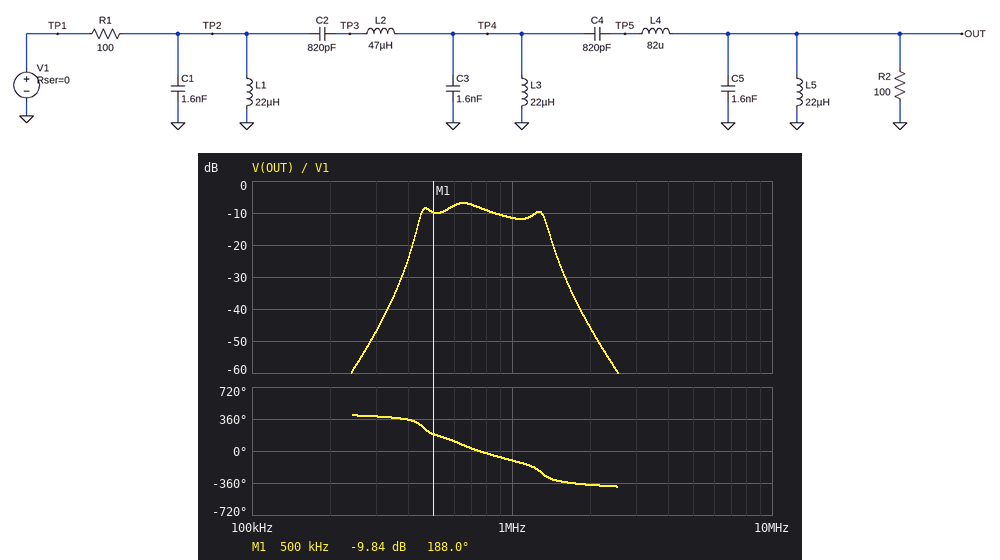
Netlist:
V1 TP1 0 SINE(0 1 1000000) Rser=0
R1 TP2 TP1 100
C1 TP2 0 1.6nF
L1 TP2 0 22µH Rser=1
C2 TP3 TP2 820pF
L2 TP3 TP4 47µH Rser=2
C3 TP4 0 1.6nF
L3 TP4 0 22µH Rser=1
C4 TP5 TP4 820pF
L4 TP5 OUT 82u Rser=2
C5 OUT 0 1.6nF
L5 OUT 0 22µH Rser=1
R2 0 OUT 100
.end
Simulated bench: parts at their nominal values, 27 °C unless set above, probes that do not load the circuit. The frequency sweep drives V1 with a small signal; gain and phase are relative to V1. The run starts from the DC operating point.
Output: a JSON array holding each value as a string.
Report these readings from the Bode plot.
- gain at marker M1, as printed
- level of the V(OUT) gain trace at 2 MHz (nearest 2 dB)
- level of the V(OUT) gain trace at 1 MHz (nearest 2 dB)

["-9.84 dB", "-46 dB", "-12 dB"]
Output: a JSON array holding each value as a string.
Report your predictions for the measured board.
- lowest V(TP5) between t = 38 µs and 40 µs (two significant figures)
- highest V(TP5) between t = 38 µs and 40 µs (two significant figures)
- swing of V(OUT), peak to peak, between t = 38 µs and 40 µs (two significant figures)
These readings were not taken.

["-1.4 V", "1.4 V", "530 mV"]
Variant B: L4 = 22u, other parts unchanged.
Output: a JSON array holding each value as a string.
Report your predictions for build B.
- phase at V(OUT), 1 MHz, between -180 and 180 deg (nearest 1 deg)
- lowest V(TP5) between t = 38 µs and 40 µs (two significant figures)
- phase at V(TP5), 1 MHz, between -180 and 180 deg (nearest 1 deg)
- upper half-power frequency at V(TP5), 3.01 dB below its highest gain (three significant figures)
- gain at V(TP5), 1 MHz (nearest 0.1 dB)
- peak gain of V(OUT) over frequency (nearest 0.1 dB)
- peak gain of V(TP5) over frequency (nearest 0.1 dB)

["-42 deg", "-720 mV", "24 deg", "1.87 MHz", "-2.8 dB", "-6.5 dB", "-2.6 dB"]
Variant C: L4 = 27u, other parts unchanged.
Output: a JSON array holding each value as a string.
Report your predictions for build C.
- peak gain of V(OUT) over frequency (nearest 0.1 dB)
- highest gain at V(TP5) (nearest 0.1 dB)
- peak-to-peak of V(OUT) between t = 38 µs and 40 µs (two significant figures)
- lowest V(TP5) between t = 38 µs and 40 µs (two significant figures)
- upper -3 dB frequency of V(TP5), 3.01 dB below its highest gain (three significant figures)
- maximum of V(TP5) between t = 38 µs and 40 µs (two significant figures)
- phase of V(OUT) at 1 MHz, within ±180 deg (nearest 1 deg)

["-6.4 dB", "0.7 dB", "950 mV", "-860 mV", "1.72 MHz", "860 mV", "-50 deg"]
